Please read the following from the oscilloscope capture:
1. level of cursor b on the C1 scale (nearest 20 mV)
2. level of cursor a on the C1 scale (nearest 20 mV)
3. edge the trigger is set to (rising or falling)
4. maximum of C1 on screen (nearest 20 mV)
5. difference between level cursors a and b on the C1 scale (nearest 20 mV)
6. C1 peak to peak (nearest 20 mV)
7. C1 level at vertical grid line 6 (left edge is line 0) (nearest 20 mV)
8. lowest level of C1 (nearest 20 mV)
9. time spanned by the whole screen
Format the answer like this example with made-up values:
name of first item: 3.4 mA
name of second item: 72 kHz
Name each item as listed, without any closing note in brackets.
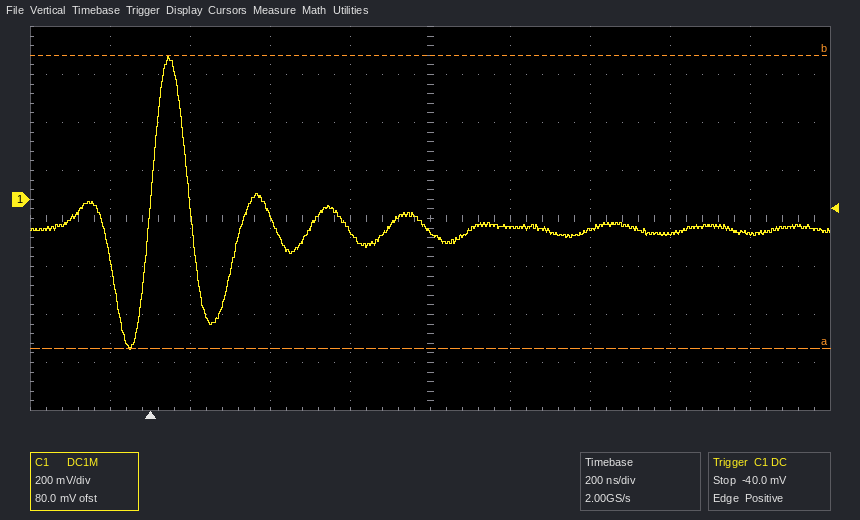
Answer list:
level of cursor b on the C1 scale: 600 mV
level of cursor a on the C1 scale: -620 mV
edge the trigger is set to: rising
maximum of C1 on screen: 600 mV
difference between level cursors a and b on the C1 scale: 1.22 V
C1 peak to peak: 1.22 V
C1 level at vertical grid line 6 (left edge is line 0): -120 mV
lowest level of C1: -620 mV
time spanned by the whole screen: 2 µs
